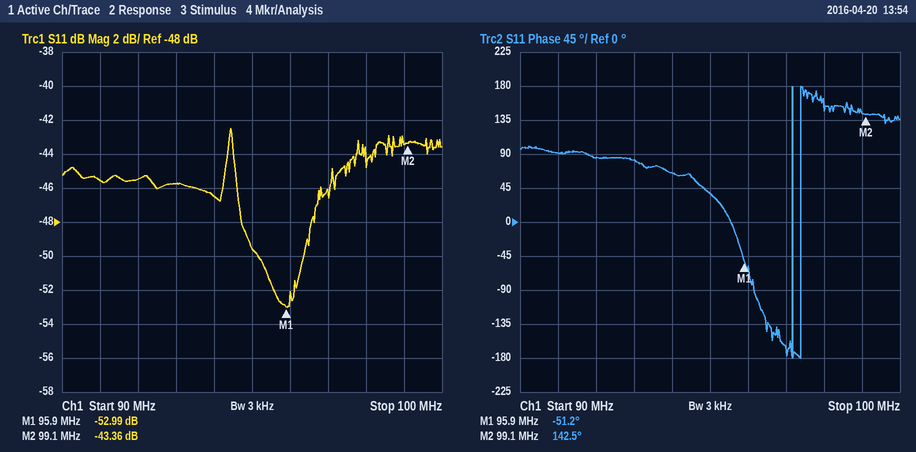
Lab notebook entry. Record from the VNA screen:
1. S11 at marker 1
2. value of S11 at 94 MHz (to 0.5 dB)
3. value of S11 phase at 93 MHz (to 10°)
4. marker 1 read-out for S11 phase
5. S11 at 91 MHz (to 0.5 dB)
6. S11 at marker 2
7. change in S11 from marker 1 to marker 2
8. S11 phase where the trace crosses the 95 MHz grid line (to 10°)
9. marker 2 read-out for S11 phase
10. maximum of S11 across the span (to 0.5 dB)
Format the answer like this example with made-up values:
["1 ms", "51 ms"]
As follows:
["-52.99 dB", "-46.5 dB", "80°", "-51.2°", "-45.5 dB", "-43.36 dB", "9.63 dB", "40°", "142.5°", "-42.5 dB"]
